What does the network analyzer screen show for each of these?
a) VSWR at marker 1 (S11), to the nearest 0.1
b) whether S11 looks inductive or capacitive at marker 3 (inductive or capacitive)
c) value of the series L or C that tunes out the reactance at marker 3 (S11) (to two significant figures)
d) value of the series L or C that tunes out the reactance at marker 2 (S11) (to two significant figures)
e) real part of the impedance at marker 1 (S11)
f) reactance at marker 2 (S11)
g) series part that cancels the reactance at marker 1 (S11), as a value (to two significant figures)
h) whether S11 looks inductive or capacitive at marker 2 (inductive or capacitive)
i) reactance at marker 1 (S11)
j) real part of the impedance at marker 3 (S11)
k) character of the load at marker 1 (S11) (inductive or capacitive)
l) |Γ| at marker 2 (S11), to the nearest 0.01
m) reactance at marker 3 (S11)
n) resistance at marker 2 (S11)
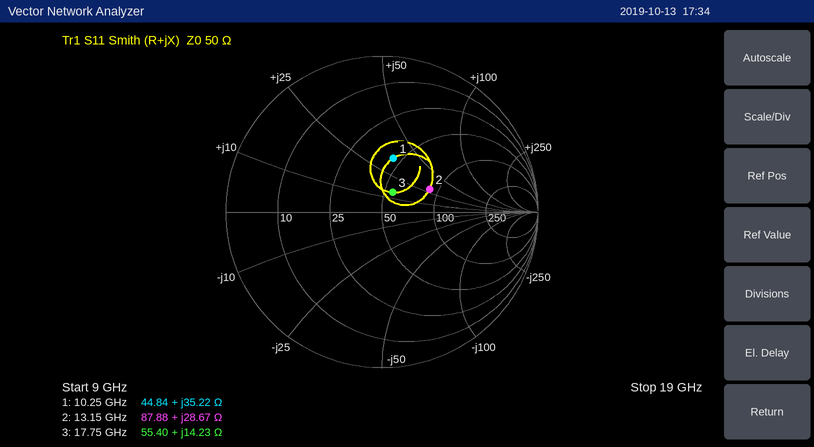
2.1
inductive
630 fF
420 fF
44.84 Ω
+28.67 Ω
440 fF
inductive
+35.22 Ω
55.40 Ω
inductive
0.34
+14.23 Ω
87.88 Ω
